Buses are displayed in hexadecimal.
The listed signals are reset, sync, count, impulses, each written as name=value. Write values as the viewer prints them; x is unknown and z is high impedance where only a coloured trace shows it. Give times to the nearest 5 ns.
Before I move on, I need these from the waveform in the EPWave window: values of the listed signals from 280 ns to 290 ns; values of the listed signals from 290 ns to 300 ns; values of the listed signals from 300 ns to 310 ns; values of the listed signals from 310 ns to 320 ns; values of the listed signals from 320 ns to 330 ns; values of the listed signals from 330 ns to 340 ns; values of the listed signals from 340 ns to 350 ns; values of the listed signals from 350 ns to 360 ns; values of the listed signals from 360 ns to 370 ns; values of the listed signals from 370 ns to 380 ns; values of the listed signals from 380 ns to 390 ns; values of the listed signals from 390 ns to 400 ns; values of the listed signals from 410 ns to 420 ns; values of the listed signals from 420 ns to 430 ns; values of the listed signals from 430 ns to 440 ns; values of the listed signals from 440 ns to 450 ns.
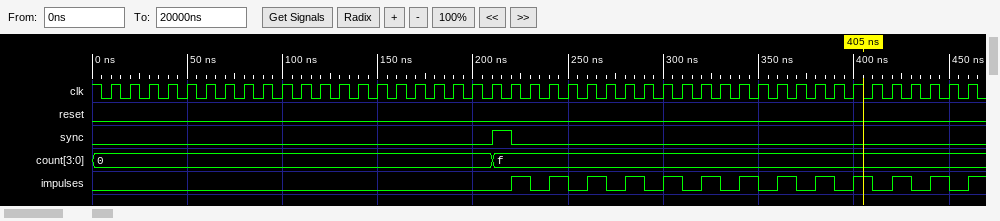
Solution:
reset=0, sync=0, count=f, impulses=1
reset=0, sync=0, count=f, impulses=0
reset=0, sync=0, count=f, impulses=1
reset=0, sync=0, count=f, impulses=0
reset=0, sync=0, count=f, impulses=1
reset=0, sync=0, count=f, impulses=0
reset=0, sync=0, count=f, impulses=1
reset=0, sync=0, count=f, impulses=0
reset=0, sync=0, count=f, impulses=1
reset=0, sync=0, count=f, impulses=0
reset=0, sync=0, count=f, impulses=1
reset=0, sync=0, count=f, impulses=0
reset=0, sync=0, count=f, impulses=0
reset=0, sync=0, count=f, impulses=1
reset=0, sync=0, count=f, impulses=0
reset=0, sync=0, count=f, impulses=1
